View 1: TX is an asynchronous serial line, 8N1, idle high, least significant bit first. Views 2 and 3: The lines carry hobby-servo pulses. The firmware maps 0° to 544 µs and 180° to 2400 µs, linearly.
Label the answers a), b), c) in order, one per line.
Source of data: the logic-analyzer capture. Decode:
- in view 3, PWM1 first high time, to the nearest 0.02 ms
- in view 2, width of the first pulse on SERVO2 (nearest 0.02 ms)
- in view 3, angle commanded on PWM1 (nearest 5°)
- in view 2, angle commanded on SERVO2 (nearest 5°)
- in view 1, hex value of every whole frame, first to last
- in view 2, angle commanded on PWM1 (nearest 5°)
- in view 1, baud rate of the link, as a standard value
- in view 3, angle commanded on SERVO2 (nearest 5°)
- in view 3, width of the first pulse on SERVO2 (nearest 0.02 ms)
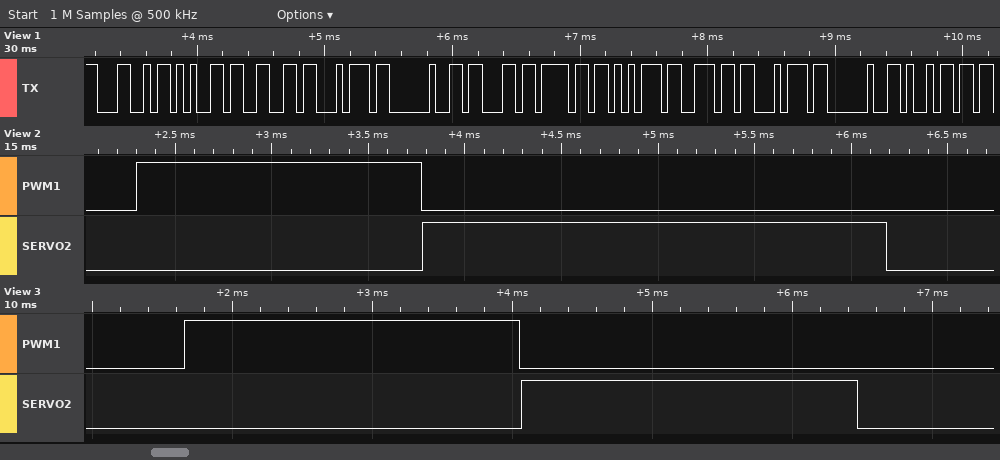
a) 2.40 ms
b) 2.40 ms
c) 180°
d) 180°
e) 0x4C 0x65 0x66 0x74 0x20 0x63 0x6F 0x75 0x6E 0x74 0x20 0x69
f) 90°
g) 19200 baud
h) 180°
i) 2.40 ms
